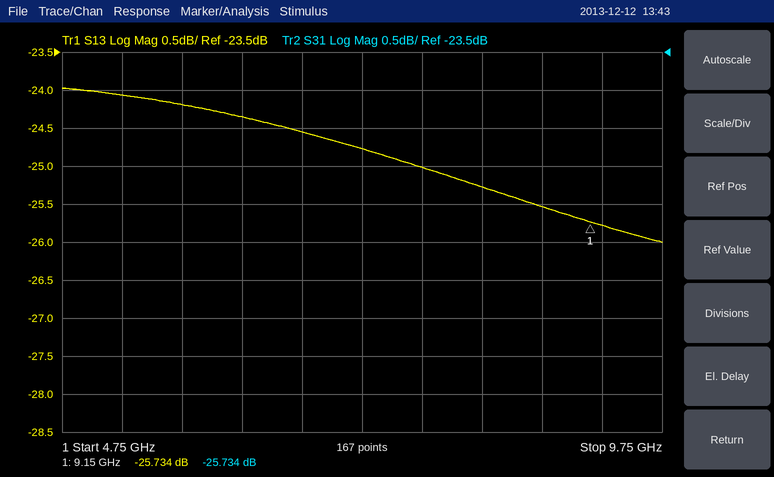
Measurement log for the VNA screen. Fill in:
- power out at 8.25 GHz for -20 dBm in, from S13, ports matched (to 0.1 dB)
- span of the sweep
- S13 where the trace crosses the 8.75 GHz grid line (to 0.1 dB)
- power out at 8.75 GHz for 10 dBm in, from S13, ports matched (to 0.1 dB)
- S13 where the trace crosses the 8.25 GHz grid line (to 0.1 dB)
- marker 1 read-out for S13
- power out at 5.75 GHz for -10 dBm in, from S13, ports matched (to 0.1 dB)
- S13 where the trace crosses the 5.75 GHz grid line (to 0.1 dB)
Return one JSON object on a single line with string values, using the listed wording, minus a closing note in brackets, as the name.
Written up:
{"power out at 8.25 GHz for -20 dBm in, from S13, ports matched": "-45.3 dBm", "span of the sweep": "5 GHz", "S13 where the trace crosses the 8.75 GHz grid line": "-25.5 dB", "power out at 8.75 GHz for 10 dBm in, from S13, ports matched": "-15.5 dBm", "S13 where the trace crosses the 8.25 GHz grid line": "-25.3 dB", "marker 1 read-out for S13": "-25.734 dB", "power out at 5.75 GHz for -10 dBm in, from S13, ports matched": "-34.2 dBm", "S13 where the trace crosses the 5.75 GHz grid line": "-24.2 dB"}
